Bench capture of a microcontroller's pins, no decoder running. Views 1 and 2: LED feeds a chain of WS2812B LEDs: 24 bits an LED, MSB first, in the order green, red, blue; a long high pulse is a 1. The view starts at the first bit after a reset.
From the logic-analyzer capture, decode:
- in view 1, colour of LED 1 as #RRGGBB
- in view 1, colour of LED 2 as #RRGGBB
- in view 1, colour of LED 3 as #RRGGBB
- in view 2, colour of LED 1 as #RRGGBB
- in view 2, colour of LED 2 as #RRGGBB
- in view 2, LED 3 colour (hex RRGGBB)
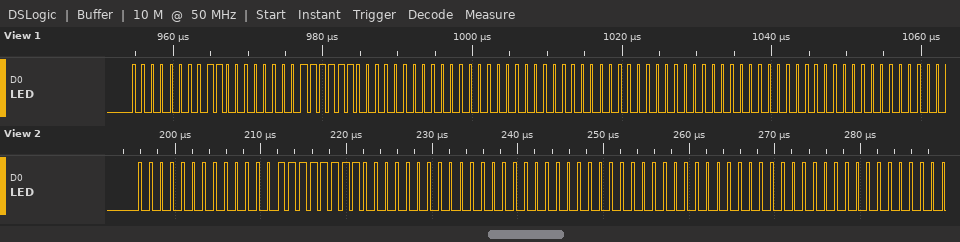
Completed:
#C0003F
#000000
#000000
#0700F8
#000000
#000000
